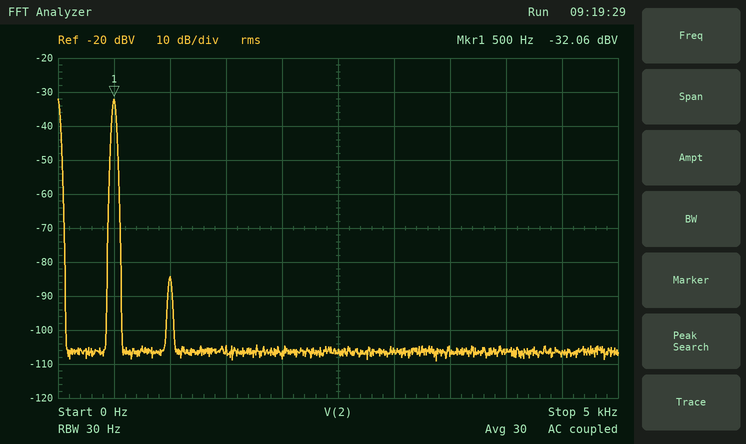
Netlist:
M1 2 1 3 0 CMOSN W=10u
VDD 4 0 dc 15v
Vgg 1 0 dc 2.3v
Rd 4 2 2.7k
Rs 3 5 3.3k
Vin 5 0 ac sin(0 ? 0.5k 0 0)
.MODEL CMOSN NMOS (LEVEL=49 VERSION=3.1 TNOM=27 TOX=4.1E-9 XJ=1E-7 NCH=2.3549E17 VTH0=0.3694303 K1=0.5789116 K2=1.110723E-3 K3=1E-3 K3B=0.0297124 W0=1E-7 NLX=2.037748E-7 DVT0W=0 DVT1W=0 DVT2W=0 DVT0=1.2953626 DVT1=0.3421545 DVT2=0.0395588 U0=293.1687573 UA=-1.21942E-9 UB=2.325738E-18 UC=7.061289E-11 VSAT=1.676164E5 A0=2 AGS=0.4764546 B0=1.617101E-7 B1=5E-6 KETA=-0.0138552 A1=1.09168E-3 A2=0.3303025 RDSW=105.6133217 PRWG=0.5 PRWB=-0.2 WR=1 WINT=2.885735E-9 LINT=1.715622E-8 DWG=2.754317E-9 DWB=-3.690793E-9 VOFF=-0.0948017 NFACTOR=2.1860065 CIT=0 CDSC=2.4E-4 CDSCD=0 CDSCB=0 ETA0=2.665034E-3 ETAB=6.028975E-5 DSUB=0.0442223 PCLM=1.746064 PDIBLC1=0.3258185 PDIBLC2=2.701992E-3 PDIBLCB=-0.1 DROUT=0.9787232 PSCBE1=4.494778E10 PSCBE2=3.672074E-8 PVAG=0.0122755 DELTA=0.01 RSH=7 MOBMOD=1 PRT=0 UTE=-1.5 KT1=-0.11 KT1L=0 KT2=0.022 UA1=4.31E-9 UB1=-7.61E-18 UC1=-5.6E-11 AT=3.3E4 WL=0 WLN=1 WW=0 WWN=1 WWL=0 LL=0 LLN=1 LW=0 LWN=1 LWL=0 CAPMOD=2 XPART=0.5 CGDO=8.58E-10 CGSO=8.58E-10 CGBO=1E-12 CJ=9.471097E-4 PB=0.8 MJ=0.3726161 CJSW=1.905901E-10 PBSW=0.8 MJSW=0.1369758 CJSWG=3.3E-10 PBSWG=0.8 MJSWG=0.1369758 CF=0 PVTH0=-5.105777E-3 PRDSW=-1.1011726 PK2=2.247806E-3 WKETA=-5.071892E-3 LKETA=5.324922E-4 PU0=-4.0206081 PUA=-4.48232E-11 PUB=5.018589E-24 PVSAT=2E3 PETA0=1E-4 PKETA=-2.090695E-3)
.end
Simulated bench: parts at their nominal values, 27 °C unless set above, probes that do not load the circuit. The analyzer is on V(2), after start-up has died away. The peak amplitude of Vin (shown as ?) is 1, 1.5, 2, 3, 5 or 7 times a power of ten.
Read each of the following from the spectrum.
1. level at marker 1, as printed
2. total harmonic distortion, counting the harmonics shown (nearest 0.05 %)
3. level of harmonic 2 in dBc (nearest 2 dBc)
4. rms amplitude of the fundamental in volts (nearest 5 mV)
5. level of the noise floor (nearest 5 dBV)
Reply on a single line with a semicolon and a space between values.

-32.06 dBV; 0.25 %; -52 dBc; 25 mV; -105 dBV
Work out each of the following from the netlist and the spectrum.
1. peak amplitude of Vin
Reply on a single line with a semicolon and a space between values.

70 mV
